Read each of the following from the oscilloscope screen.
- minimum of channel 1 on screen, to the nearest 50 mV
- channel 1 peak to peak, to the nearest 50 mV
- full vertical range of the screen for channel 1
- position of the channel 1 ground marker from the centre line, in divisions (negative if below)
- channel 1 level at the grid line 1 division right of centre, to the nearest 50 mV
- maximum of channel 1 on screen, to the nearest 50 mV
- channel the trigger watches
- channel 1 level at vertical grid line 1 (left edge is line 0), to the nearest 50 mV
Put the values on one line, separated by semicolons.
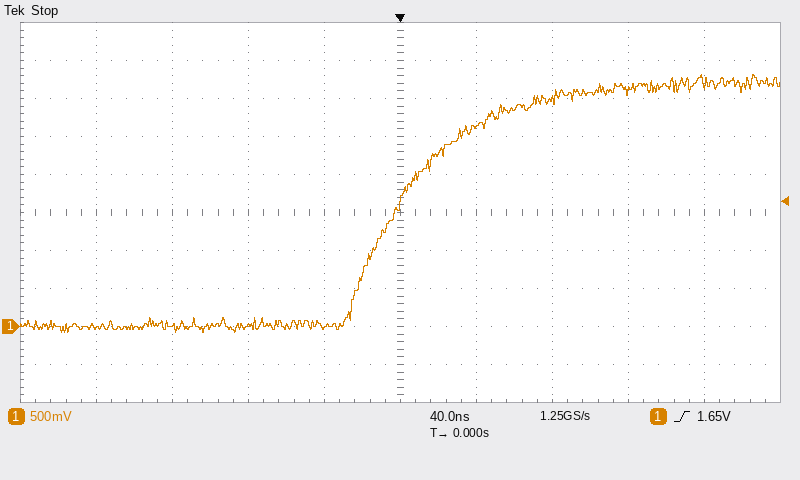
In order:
-100 mV; 3.40 V; 5 V; -3.0 div; 2.65 V; 3.30 V; channel 1; 0 mV
